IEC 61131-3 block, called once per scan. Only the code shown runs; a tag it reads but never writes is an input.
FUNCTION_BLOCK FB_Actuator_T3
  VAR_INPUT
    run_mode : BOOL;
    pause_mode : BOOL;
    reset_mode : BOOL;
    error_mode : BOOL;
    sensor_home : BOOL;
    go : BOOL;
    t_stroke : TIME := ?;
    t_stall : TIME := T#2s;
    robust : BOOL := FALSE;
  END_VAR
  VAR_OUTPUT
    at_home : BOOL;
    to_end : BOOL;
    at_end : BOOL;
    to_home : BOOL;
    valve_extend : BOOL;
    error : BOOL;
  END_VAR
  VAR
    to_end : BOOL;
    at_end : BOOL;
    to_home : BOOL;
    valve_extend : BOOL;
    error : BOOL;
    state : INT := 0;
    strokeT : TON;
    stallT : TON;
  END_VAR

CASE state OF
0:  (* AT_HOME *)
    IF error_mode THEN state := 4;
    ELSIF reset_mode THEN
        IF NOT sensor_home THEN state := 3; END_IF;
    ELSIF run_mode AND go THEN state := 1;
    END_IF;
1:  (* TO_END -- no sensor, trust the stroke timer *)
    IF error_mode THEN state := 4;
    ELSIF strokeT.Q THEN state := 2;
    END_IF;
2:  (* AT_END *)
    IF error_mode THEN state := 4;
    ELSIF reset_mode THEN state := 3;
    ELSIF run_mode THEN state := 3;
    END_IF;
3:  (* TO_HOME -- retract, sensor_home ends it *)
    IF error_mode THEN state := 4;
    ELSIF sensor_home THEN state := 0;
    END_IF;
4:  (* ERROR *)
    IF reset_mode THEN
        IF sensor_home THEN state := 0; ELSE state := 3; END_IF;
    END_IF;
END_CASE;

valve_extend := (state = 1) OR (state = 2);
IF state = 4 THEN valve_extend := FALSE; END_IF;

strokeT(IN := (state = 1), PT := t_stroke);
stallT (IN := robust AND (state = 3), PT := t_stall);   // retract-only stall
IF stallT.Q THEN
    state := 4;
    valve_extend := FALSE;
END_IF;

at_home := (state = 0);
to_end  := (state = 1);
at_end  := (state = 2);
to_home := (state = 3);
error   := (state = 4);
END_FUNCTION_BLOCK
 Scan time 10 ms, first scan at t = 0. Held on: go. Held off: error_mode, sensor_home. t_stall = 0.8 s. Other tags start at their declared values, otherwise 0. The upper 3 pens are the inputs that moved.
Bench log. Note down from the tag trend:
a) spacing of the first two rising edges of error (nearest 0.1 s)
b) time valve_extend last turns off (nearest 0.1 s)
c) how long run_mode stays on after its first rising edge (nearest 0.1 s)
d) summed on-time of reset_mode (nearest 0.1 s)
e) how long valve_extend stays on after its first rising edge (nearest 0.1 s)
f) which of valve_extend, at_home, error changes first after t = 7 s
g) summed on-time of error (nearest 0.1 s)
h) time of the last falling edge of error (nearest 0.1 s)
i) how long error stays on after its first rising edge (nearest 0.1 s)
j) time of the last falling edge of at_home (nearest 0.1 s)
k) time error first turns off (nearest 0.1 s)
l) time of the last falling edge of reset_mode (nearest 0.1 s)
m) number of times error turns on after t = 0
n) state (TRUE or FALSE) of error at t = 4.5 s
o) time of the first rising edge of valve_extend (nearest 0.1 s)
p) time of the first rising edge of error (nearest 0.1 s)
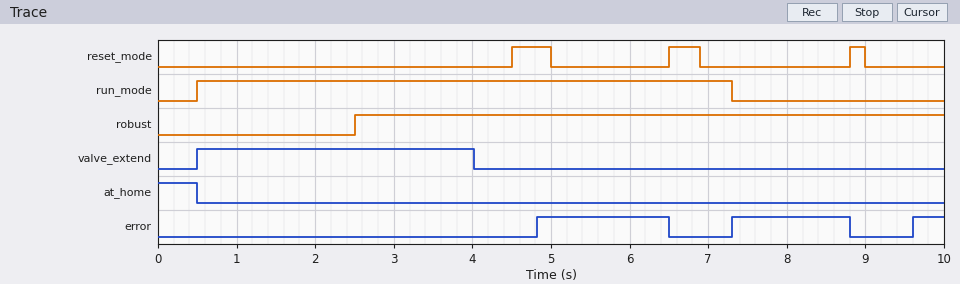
2.5 s
4.0 s
6.8 s
1.1 s
3.5 s
error
3.6 s
8.8 s
1.7 s
0.5 s
6.5 s
9.0 s
3
FALSE
0.5 s
4.8 s
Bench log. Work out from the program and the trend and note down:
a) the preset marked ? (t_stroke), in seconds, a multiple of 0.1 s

3.5 s
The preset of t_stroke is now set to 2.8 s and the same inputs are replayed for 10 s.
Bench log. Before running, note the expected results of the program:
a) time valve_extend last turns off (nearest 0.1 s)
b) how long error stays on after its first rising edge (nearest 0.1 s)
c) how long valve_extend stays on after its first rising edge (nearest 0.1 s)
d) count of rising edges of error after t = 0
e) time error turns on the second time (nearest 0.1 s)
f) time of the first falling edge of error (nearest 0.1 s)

3.3 s
0.4 s
2.8 s
4
5.3 s
4.5 s
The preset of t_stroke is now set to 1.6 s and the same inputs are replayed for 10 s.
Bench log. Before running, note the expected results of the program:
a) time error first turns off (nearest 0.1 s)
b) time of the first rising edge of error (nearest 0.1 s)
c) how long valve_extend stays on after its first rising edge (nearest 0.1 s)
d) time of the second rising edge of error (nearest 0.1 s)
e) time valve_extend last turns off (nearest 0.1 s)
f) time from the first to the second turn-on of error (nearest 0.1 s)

4.5 s
3.3 s
1.6 s
5.3 s
2.1 s
2.0 s
